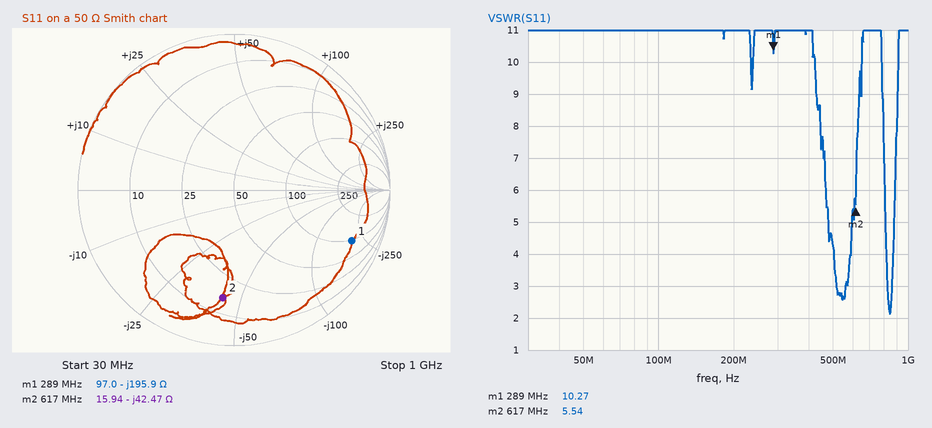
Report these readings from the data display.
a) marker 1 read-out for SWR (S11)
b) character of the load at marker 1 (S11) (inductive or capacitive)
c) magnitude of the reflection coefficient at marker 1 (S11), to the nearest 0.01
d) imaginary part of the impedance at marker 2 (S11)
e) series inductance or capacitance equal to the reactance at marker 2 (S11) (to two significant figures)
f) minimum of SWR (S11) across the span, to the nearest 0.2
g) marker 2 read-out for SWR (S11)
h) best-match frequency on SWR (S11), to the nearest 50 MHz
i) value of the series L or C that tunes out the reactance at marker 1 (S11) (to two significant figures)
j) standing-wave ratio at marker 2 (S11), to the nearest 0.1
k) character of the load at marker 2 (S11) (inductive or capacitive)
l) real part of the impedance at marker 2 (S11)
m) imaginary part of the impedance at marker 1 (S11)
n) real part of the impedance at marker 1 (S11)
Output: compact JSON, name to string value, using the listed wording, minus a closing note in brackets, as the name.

{"marker 1 read-out for SWR": "10.27", "character of the load at marker 1 (S11)": "capacitive", "magnitude of the reflection coefficient at marker 1 (S11), to the nearest 0.01": "0.82", "imaginary part of the impedance at marker 2": "-42.47 Ω", "series inductance or capacitance equal to the reactance at marker 2 (S11)": "6.1 pF", "minimum of SWR (S11) across the span, to the nearest 0.2": "2.2", "marker 2 read-out for SWR": "5.54", "best-match frequency on SWR (S11), to the nearest 50 MHz": "850 MHz", "value of the series L or C that tunes out the reactance at marker 1 (S11)": "110 nH", "standing-wave ratio at marker 2 (S11), to the nearest 0.1": "5.5", "character of the load at marker 2 (S11)": "capacitive", "real part of the impedance at marker 2": "15.94 Ω", "imaginary part of the impedance at marker 1": "-195.9 Ω", "real part of the impedance at marker 1": "97.0 Ω"}
